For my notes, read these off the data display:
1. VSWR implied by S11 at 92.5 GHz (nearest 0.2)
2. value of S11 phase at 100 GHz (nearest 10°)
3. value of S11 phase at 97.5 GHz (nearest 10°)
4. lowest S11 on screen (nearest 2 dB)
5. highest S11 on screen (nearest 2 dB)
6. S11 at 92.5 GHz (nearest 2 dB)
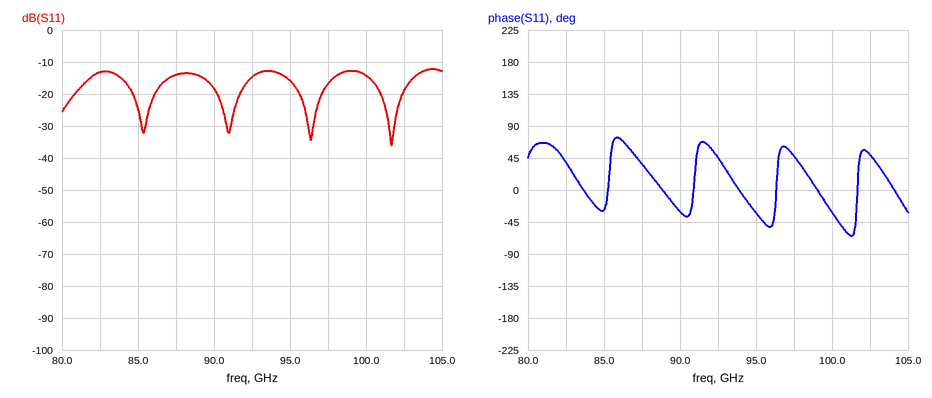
1.4
-30°
50°
-36 dB
-12 dB
-14 dB
